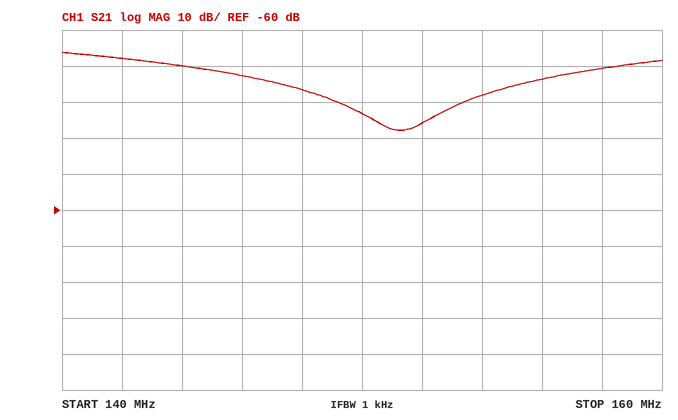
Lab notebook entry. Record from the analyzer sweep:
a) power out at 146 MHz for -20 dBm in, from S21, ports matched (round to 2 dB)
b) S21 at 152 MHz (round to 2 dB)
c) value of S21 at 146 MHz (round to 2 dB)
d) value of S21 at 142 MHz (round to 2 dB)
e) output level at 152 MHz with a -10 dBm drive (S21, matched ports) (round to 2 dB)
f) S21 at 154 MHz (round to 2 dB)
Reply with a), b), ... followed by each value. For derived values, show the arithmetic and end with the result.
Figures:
a) -20 dBm + (-22 dB) = -42 dBm
b) -36 dB
c) -22 dB
d) -18 dB
e) -10 dBm + (-36 dB) = -46 dBm
f) -28 dB
